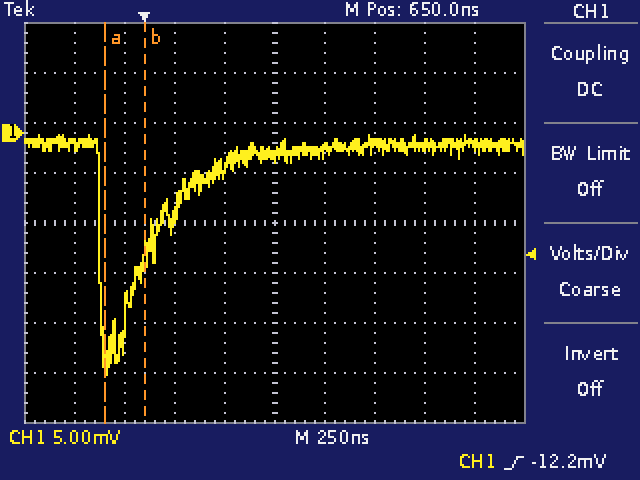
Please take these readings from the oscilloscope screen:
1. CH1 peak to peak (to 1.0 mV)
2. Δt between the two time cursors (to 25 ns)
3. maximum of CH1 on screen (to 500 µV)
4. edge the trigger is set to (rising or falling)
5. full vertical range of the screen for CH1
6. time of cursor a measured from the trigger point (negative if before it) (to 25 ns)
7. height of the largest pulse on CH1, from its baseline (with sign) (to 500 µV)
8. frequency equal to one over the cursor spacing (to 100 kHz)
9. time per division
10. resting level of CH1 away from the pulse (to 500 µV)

24.0 mV
200 ns
0.0 mV
rising
40 mV
-200 ns
-23.0 mV
5.0 MHz
250 ns
-1.0 mV
